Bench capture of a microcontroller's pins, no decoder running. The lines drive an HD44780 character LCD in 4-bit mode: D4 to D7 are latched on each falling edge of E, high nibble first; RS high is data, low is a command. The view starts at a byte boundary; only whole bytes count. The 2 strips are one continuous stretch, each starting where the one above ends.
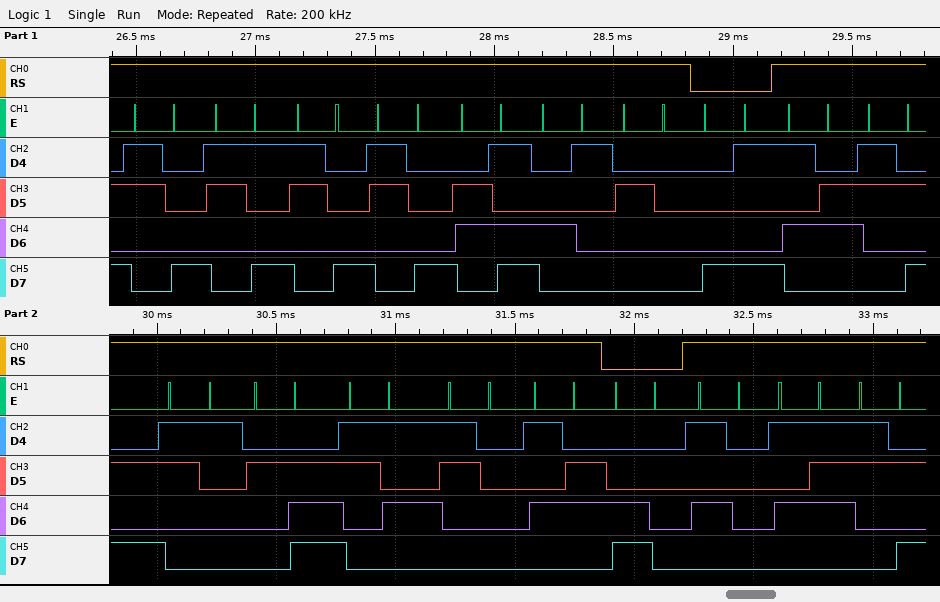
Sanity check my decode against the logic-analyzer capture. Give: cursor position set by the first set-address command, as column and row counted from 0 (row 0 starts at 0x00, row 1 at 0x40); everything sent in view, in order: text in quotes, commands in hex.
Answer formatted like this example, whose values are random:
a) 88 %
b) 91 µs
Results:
a) column 9, row 0
b) "8988mA " 0x89 "V:1.50V" 0xC0 "PW:"
